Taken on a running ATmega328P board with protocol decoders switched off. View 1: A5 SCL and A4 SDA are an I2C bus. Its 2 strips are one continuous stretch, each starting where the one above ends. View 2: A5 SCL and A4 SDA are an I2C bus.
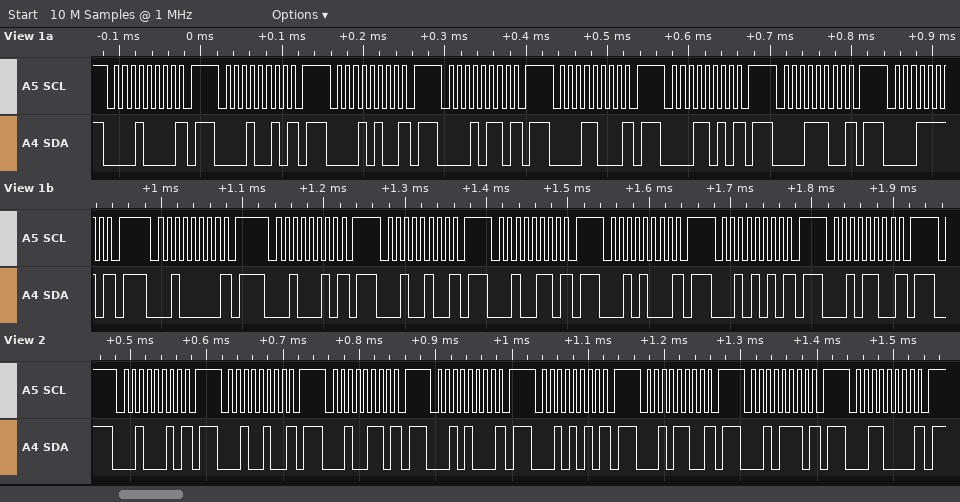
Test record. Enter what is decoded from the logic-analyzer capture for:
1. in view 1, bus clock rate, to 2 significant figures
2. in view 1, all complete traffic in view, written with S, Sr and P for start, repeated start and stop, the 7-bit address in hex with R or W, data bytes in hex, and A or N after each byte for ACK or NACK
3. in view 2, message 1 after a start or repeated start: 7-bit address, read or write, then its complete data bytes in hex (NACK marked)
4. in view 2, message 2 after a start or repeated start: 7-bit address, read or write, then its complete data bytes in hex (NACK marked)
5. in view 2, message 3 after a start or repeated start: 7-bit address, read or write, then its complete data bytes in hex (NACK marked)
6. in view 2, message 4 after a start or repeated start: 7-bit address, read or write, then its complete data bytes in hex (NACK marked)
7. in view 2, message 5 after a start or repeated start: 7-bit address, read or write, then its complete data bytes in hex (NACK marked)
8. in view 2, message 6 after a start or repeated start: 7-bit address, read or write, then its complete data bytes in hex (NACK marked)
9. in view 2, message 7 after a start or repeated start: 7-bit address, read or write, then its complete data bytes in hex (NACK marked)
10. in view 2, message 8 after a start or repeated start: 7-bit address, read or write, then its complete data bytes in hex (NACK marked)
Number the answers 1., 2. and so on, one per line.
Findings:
1. 100 kHz
2. S 08W N P S 09W N P S 0AW N P S 0BW N P S 0CW N P S 0DW N P S 0EW N P S 0FW N P S 10W N P S 11W N P S 12W N P S 13W N P S 14W N P S 15W N P S 16W N P
3. 0x11 write NACK
4. 0x12 write NACK
5. 0x13 write NACK
6. 0x14 write NACK
7. 0x15 write NACK
8. 0x16 write NACK
9. 0x17 write NACK
10. 0x18 write NACK
